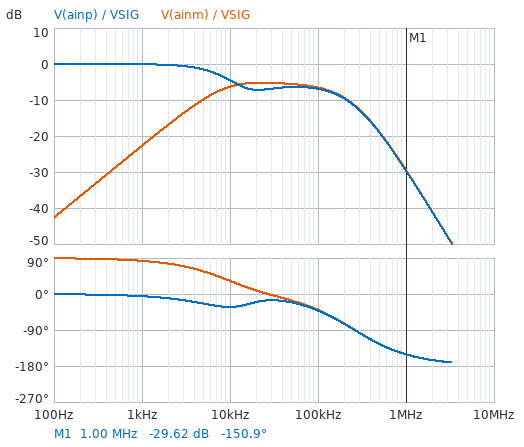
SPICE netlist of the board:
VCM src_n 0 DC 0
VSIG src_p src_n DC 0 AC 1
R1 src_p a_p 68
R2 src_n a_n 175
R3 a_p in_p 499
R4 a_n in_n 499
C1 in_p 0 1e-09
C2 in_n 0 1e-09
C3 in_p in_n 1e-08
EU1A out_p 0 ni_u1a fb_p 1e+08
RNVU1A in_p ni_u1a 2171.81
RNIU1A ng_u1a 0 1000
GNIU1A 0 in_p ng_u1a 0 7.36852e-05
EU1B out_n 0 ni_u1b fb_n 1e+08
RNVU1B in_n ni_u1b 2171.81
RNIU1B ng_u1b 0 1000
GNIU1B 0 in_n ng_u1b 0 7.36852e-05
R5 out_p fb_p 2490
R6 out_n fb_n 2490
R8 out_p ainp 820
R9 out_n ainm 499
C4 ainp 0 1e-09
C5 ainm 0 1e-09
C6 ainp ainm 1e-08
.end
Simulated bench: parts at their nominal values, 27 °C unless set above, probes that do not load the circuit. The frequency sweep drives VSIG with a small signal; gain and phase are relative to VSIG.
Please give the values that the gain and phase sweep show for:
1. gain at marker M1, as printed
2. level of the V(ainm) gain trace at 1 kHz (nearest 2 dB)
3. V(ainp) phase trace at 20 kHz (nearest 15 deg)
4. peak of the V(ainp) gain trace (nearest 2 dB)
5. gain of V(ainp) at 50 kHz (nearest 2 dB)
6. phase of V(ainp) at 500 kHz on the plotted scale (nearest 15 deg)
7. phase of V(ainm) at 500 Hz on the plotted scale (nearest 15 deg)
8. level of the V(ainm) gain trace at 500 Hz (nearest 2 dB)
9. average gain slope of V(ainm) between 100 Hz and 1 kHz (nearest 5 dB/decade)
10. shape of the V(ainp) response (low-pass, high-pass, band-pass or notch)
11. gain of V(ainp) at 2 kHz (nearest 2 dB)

-29.62 dB
-22 dB
-15 deg
0 dB
-6 dB
-120 deg
90 deg
-28 dB
20 dB/decade
low-pass
0 dB
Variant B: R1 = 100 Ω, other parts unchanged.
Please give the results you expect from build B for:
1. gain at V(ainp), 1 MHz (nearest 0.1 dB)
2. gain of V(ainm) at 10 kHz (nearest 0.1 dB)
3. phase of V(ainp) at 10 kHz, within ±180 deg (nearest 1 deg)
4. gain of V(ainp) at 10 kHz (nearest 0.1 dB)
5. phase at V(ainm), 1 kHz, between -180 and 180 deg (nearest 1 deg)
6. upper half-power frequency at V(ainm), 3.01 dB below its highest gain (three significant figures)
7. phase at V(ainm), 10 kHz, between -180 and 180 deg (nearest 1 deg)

-30.1 dB
-6.4 dB
-33 deg
-4.6 dB
83 deg
157 kHz
32 deg
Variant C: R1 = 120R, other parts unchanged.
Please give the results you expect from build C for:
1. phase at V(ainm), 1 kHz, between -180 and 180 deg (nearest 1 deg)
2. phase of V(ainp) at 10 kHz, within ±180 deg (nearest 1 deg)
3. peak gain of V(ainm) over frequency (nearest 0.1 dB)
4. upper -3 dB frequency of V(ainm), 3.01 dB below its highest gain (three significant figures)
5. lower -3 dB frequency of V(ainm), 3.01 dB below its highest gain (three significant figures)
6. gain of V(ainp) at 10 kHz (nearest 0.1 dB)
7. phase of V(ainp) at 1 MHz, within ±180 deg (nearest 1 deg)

83 deg
-34 deg
-5.5 dB
155 kHz
6.30 kHz
-4.7 dB
-152 deg
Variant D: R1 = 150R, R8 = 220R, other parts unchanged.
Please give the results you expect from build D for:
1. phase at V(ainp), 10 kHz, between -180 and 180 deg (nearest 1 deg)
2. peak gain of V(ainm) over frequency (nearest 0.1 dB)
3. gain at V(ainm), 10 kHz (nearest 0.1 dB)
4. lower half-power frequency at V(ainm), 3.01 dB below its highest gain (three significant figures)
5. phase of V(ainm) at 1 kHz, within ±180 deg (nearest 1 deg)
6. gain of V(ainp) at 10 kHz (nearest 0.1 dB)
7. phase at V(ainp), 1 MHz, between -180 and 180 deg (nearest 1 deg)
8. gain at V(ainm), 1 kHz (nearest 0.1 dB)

-24 deg
-4.3 dB
-5.7 dB
7.10 kHz
84 deg
-2.3 dB
-139 deg
-22.7 dB
